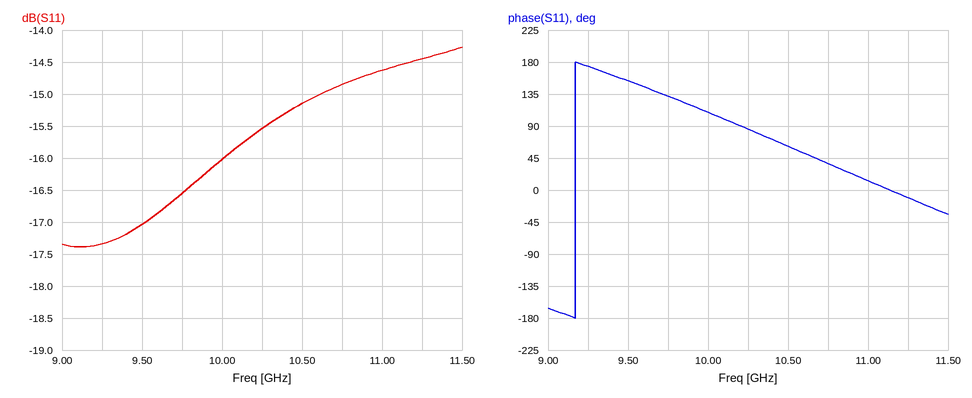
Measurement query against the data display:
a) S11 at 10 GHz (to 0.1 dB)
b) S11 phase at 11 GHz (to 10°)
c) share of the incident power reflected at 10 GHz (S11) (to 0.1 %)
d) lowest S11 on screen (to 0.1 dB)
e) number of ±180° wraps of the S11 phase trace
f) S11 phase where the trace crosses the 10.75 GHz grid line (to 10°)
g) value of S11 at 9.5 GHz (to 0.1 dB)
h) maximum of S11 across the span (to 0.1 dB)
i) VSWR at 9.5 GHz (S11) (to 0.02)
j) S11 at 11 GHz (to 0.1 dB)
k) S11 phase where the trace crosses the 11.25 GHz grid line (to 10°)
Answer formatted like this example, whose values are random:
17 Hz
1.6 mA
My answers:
-16.0 dB
10°
2.5 %
-17.4 dB
1
40°
-17.0 dB
-14.3 dB
1.32
-14.6 dB
-10°
